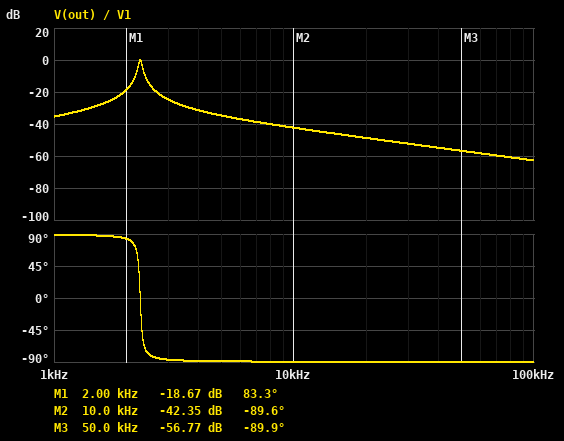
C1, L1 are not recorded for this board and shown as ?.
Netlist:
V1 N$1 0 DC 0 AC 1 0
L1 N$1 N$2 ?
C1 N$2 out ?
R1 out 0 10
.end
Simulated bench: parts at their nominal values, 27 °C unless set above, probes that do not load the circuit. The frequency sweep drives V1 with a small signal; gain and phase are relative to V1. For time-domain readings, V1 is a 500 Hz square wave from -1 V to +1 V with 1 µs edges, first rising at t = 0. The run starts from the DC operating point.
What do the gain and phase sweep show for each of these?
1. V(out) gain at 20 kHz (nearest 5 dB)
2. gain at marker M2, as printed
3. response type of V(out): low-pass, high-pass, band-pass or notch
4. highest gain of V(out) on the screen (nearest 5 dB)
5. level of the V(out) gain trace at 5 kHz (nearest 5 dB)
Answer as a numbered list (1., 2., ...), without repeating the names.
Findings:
1. -50 dB
2. -42.35 dB
3. band-pass
4. 0 dB
5. -35 dB
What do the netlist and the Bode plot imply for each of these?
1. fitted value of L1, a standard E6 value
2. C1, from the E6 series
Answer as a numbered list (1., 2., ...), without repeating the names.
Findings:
1. 22 mH
2. 220 nF
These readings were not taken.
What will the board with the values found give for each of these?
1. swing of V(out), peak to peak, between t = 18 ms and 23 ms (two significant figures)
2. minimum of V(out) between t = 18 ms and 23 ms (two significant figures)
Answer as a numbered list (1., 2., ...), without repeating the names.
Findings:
1. 110 mV
2. -54 mV
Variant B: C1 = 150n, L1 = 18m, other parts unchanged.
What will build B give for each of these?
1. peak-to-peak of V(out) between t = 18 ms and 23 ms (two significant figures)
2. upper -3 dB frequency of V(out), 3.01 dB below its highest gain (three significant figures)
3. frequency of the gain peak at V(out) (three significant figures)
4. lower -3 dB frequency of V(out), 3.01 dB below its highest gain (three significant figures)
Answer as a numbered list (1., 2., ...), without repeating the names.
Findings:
1. 65 mV
2. 3.11 kHz
3. 3.06 kHz
4. 3.02 kHz
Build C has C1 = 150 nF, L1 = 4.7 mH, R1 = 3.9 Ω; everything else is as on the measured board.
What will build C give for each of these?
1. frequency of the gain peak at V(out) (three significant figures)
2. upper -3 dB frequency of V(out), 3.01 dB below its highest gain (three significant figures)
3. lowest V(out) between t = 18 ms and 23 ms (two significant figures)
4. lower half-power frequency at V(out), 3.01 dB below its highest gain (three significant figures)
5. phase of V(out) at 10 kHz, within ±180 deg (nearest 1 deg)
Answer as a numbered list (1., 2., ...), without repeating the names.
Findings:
1. 5.99 kHz
2. 6.06 kHz
3. -26 mV
4. 5.93 kHz
5. -89 deg
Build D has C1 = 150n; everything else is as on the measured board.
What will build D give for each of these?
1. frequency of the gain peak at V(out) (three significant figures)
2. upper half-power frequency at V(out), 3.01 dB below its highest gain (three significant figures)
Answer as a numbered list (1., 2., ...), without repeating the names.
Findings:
1. 2.77 kHz
2. 2.81 kHz
